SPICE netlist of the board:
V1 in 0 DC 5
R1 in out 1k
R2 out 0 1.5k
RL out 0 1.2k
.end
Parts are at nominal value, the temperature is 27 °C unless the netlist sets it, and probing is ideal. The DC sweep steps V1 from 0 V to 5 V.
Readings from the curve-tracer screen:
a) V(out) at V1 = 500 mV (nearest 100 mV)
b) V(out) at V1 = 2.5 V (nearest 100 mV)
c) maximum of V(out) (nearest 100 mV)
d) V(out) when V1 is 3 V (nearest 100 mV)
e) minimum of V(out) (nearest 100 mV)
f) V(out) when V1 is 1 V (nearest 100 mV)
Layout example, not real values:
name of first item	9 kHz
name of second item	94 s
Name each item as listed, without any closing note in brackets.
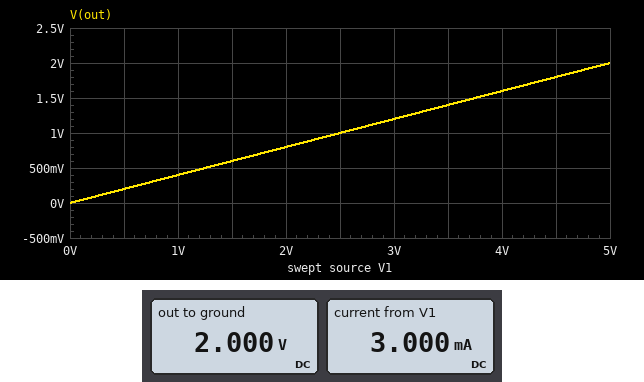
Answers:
V(out) at V1 = 500 mV	200 mV
V(out) at V1 = 2.5 V	1.0 V
maximum of V(out)	2.0 V
V(out) when V1 is 3 V	1.2 V
minimum of V(out)	0 V
V(out) when V1 is 1 V	400 mV
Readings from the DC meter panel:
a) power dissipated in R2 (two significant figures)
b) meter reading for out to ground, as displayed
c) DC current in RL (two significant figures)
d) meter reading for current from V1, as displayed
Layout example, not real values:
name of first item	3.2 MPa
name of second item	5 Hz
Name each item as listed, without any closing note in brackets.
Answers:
power dissipated in R2	2.7 mW
meter reading for out to ground, as displayed	2.000 V
DC current in RL	1.7 mA
meter reading for current from V1, as displayed	3.000 mA
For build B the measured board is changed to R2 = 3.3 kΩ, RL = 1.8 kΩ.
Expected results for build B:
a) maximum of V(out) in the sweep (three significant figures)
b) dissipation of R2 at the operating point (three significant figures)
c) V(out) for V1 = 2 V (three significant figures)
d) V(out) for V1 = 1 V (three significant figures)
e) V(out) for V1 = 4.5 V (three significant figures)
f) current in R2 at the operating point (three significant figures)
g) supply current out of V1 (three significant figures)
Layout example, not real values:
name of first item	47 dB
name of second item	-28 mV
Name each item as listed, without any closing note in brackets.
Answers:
maximum of V(out) in the sweep	2.69 V
dissipation of R2 at the operating point	2.19 mW
V(out) for V1 = 2 V	1.08 V
V(out) for V1 = 1 V	538 mV
V(out) for V1 = 4.5 V	2.42 V
current in R2 at the operating point	815 µA
supply current out of V1	2.31 mA
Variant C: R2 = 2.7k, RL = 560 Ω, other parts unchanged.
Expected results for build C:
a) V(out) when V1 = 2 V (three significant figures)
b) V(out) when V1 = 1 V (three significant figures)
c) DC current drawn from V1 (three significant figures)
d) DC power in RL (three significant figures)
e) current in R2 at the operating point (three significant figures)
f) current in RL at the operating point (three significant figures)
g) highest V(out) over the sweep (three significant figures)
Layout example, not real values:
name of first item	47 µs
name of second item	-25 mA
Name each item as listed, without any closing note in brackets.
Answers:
V(out) when V1 = 2 V	634 mV
V(out) when V1 = 1 V	317 mV
DC current drawn from V1	3.42 mA
DC power in RL	4.48 mW
current in R2 at the operating point	587 µA
current in RL at the operating point	2.83 mA
highest V(out) over the sweep	1.58 V
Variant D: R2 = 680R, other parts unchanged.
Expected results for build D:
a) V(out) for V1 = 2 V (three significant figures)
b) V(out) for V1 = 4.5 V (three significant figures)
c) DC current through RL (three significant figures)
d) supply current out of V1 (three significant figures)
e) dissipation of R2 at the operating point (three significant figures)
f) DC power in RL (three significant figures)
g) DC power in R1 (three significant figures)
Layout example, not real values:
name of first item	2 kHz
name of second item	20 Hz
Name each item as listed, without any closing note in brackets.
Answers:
V(out) for V1 = 2 V	605 mV
V(out) for V1 = 4.5 V	1.36 V
DC current through RL	1.26 mA
supply current out of V1	3.49 mA
dissipation of R2 at the operating point	3.37 mW
DC power in RL	1.91 mW
DC power in R1	12.2 mW
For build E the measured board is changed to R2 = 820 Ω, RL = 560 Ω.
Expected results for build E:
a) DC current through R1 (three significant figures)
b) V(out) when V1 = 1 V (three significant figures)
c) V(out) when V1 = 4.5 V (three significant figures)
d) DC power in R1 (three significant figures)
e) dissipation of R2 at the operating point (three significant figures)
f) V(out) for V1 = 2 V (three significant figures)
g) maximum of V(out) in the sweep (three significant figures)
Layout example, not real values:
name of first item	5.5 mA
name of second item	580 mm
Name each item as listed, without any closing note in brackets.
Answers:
DC current through R1	3.75 mA
V(out) when V1 = 1 V	250 mV
V(out) when V1 = 4.5 V	1.12 V
DC power in R1	14.1 mW
dissipation of R2 at the operating point	1.90 mW
V(out) for V1 = 2 V	499 mV
maximum of V(out) in the sweep	1.25 V
